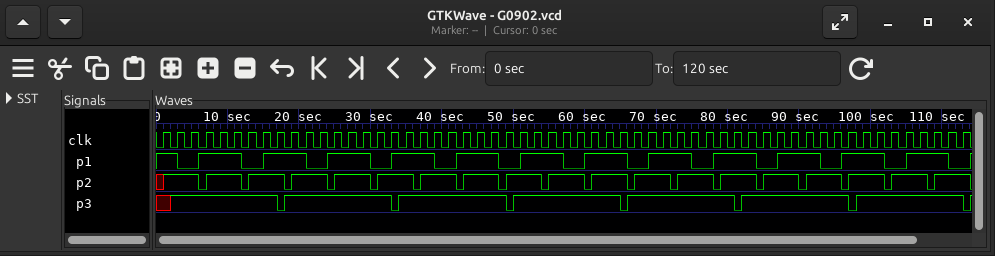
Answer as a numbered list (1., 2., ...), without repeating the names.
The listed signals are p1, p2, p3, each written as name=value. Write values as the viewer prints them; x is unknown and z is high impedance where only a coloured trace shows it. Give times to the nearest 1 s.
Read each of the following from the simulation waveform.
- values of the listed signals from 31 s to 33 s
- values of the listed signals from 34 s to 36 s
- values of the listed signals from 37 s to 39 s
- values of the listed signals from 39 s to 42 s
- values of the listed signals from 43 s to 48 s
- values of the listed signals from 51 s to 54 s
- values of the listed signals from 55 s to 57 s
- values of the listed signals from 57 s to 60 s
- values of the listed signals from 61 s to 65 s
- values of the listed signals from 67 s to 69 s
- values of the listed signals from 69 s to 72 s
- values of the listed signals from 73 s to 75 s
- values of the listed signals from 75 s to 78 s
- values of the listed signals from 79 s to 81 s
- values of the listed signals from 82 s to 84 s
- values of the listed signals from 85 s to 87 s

1. p1=0, p2=1, p3=1
2. p1=1, p2=1, p3=1
3. p1=1, p2=1, p3=1
4. p1=0, p2=1, p3=1
5. p1=1, p2=1, p3=1
6. p1=1, p2=1, p3=1
7. p1=1, p2=1, p3=1
8. p1=0, p2=1, p3=1
9. p1=1, p2=1, p3=1
10. p1=0, p2=1, p3=1
11. p1=1, p2=1, p3=1
12. p1=1, p2=1, p3=1
13. p1=0, p2=1, p3=1
14. p1=1, p2=1, p3=1
15. p1=1, p2=1, p3=1
16. p1=0, p2=1, p3=1
